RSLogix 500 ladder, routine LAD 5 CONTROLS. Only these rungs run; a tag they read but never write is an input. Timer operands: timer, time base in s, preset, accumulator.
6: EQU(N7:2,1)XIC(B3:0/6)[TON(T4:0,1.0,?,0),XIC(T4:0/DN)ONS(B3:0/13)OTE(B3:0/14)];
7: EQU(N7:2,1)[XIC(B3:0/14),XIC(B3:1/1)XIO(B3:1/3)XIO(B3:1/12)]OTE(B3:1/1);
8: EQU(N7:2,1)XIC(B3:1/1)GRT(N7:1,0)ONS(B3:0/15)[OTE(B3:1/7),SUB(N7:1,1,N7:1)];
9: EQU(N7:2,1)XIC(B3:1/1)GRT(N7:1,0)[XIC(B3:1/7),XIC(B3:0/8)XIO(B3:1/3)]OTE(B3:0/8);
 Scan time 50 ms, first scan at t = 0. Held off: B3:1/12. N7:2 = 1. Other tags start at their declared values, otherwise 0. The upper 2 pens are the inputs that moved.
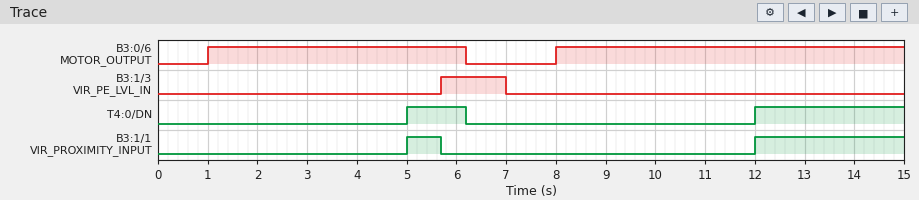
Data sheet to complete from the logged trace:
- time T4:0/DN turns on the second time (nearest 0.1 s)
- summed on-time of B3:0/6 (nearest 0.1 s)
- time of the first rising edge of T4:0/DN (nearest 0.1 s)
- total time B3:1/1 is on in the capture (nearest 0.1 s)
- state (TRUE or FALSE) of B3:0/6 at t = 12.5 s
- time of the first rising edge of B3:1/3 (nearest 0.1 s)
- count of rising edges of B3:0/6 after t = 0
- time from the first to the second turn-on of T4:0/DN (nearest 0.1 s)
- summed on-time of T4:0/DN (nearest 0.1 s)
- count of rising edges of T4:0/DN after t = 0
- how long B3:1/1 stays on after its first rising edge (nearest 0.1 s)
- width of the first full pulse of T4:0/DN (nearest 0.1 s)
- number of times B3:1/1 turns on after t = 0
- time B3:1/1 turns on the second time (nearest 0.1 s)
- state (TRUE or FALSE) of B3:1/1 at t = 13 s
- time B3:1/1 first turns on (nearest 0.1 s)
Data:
12.0 s
12.2 s
5.0 s
3.7 s
TRUE
5.7 s
2
7.0 s
4.2 s
2
0.7 s
1.2 s
2
12.0 s
TRUE
5.0 s
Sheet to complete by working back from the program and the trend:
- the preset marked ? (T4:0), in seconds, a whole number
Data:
4 s
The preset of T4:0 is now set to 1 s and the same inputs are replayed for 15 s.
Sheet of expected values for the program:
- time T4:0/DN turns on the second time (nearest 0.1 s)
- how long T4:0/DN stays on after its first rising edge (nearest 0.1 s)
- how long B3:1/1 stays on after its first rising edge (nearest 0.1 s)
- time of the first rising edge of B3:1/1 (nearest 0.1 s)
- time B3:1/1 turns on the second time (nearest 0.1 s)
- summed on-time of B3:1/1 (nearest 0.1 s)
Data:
9.0 s
4.2 s
3.7 s
2.0 s
9.0 s
9.7 s
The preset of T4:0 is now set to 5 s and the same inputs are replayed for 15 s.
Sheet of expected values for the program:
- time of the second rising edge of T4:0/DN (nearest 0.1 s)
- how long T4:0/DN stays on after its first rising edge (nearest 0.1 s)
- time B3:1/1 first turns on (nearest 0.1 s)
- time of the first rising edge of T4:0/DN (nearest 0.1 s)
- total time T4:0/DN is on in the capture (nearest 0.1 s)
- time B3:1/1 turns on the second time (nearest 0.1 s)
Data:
13.0 s
0.2 s
6.0 s
6.0 s
2.2 s
13.0 s
